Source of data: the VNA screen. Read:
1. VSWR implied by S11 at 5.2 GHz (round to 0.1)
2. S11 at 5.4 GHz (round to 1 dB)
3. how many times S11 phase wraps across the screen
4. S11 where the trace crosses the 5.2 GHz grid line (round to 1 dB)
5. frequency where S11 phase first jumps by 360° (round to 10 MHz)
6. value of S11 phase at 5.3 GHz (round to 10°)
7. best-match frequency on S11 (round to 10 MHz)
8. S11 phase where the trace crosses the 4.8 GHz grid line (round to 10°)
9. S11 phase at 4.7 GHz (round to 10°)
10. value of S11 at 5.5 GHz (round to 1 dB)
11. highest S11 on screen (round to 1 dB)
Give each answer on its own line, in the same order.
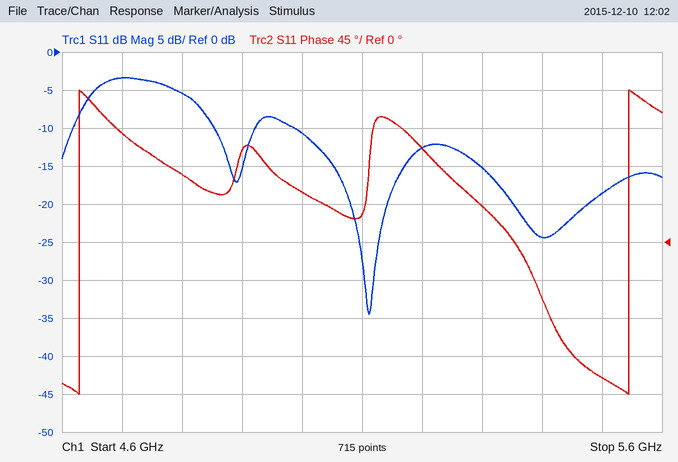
1.6
-24 dB
2
-13 dB
4.63 GHz
40°
5.11 GHz
80°
130°
-19 dB
-3 dB
